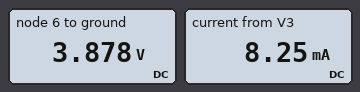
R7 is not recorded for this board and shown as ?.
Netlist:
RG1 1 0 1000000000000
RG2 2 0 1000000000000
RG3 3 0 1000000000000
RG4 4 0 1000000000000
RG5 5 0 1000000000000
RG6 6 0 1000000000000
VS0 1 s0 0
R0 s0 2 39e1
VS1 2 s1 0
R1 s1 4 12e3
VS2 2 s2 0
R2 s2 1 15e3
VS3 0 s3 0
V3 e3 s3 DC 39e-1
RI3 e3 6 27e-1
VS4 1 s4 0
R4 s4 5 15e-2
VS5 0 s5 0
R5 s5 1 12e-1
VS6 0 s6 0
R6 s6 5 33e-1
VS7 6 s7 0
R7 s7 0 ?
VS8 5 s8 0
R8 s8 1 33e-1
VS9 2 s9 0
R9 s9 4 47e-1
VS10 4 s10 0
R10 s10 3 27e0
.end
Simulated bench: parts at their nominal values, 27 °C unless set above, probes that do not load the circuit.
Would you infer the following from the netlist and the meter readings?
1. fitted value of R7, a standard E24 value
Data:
470 Ω
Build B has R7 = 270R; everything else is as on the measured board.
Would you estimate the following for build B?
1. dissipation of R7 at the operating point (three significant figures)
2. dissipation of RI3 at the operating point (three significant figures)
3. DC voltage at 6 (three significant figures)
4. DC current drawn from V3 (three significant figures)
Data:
55.2 mW
552 µW
3.86 V
14.3 mA
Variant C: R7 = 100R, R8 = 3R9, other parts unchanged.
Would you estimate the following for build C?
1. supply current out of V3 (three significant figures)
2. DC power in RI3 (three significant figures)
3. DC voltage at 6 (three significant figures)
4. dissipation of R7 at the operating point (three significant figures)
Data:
38.0 mA
3.89 mW
3.80 V
144 mW
